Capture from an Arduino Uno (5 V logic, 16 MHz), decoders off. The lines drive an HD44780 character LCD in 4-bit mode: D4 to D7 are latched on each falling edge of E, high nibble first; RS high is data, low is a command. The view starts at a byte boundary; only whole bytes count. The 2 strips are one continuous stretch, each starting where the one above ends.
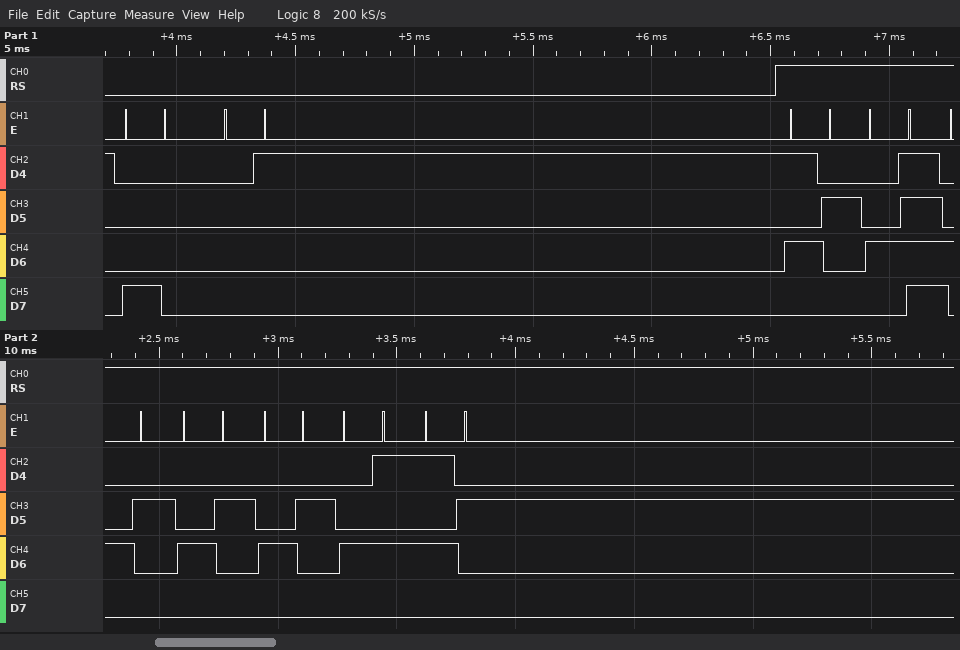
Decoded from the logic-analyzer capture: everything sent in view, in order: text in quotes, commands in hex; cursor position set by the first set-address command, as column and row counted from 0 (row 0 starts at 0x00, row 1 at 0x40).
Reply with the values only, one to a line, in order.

0x80 0x01 "ROBBBER"
column 0, row 0
